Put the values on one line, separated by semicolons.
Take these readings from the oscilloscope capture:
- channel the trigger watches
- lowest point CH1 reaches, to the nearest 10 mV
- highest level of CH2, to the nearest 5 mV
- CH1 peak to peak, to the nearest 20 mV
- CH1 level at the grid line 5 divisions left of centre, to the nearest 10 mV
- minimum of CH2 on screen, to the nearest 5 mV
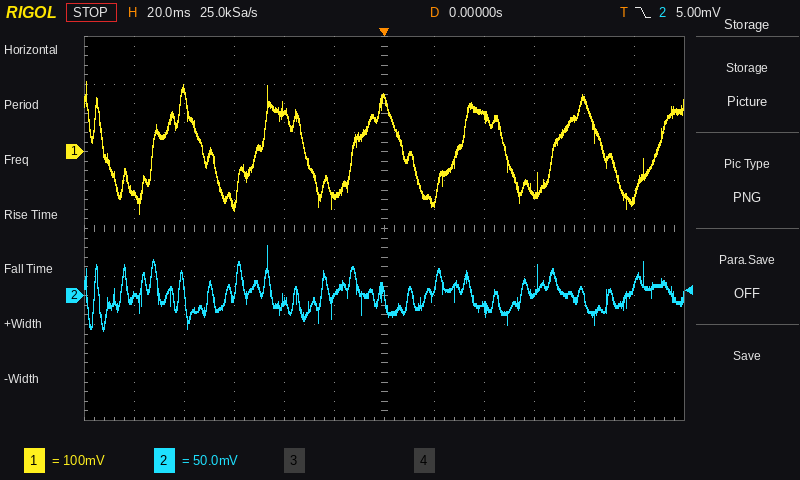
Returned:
CH2; -130 mV; 50 mV; 280 mV; -90 mV; -35 mV
